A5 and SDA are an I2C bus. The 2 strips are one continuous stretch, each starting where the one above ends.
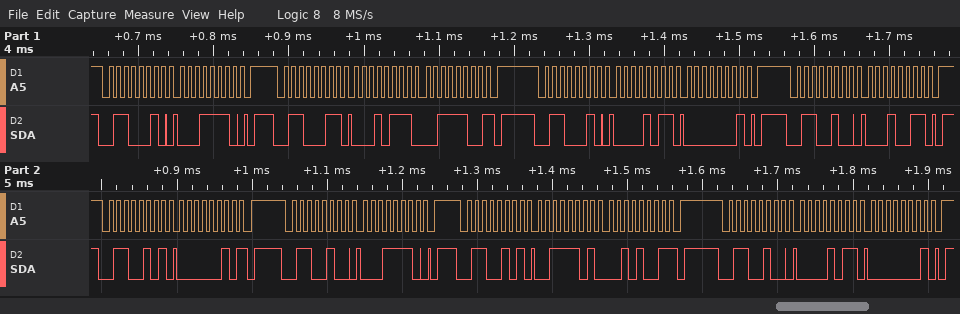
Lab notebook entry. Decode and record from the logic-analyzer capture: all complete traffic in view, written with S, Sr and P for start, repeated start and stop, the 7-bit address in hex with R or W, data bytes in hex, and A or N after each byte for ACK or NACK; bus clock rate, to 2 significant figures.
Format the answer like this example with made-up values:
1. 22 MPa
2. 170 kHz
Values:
1. S 31W A 1E A P S 31R A 17 A 3C N P S 31W A 0B A 01 A P S 32W A 13 A P S 32R A 02 N P S 32W A 1E A P S 32R A 3D A 29 N P S 32W A 0B A 01 A P
2. 100 kHz
